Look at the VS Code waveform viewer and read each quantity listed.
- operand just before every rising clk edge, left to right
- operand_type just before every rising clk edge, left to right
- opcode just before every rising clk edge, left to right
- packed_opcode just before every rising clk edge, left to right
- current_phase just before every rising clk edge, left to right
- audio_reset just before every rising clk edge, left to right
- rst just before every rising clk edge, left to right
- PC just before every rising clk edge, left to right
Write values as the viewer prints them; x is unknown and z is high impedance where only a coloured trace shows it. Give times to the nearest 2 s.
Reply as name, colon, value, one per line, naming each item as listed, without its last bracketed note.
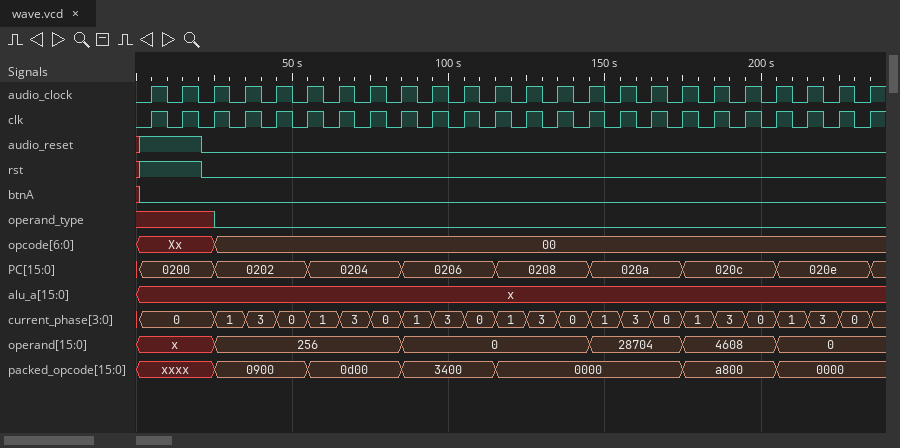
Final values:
operand just before every rising clk edge, left to right: x, x, x, 256, 256, 256, 256, 256, 256, 0, 0, 0, 0, 0, 0, 28704, 28704, 28704, 4608, 4608, 4608, 0, 0, 0
operand_type just before every rising clk edge, left to right: x x x 0 0 0 0 0 0 0 0 0 0 0 0 0 0 0 0 0 0 0 0 0
opcode just before every rising clk edge, left to right: Xx, Xx, Xx, 00, 00, 00, 00, 00, 00, 00, 00, 00, 00, 00, 00, 00, 00, 00, 00, 00, 00, 00, 00, 00
packed_opcode just before every rising clk edge, left to right: xxxx, xxxx, xxxx, 0900, 0900, 0900, 0d00, 0d00, 0d00, 3400, 3400, 3400, 0000, 0000, 0000, 0000, 0000, 0000, a800, a800, a800, 0000, 0000, 0000
current_phase just before every rising clk edge, left to right: 0, 0, 0, 1, 3, 0, 1, 3, 0, 1, 3, 0, 1, 3, 0, 1, 3, 0, 1, 3, 0, 1, 3, 0
audio_reset just before every rising clk edge, left to right: 1 1 0 0 0 0 0 0 0 0 0 0 0 0 0 0 0 0 0 0 0 0 0 0
rst just before every rising clk edge, left to right: 1 1 0 0 0 0 0 0 0 0 0 0 0 0 0 0 0 0 0 0 0 0 0 0
PC just before every rising clk edge, left to right: 0200, 0200, 0200, 0202, 0202, 0202, 0204, 0204, 0204, 0206, 0206, 0206, 0208, 0208, 0208, 020a, 020a, 020a, 020c, 020c, 020c, 020e, 020e, 020e
